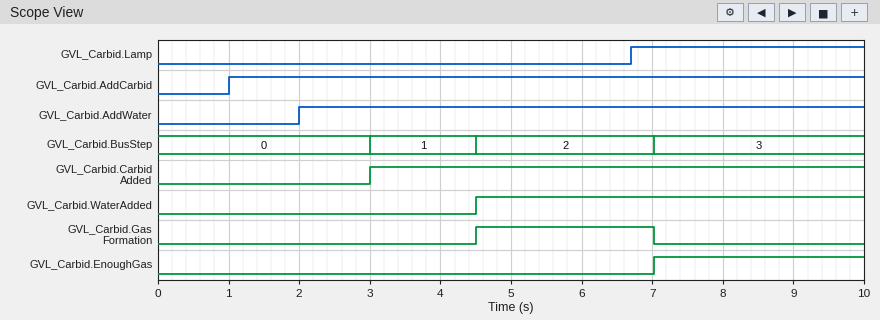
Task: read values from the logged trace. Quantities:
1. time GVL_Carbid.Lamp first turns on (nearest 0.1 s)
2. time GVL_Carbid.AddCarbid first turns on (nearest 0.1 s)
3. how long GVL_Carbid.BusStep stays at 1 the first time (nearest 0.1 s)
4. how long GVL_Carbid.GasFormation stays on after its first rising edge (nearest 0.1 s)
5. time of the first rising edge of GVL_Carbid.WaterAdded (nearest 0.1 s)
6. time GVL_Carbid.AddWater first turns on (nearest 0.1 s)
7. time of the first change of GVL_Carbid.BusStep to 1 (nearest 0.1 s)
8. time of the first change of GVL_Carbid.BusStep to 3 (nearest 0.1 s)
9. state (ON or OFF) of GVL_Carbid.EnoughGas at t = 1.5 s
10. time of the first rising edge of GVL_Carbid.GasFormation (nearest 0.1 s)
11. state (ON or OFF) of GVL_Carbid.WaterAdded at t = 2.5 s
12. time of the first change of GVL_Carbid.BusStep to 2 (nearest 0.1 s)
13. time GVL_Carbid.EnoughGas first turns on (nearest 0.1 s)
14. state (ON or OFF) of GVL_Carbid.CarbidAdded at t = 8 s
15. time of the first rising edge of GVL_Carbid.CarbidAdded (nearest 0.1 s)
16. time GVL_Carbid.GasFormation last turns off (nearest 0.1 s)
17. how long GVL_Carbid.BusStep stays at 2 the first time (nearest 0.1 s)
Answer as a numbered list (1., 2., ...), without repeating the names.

1. 6.7 s
2. 1.0 s
3. 1.5 s
4. 2.5 s
5. 4.5 s
6. 2.0 s
7. 3.0 s
8. 7.0 s
9. OFF
10. 4.5 s
11. OFF
12. 4.5 s
13. 7.0 s
14. ON
15. 3.0 s
16. 7.0 s
17. 2.5 s
